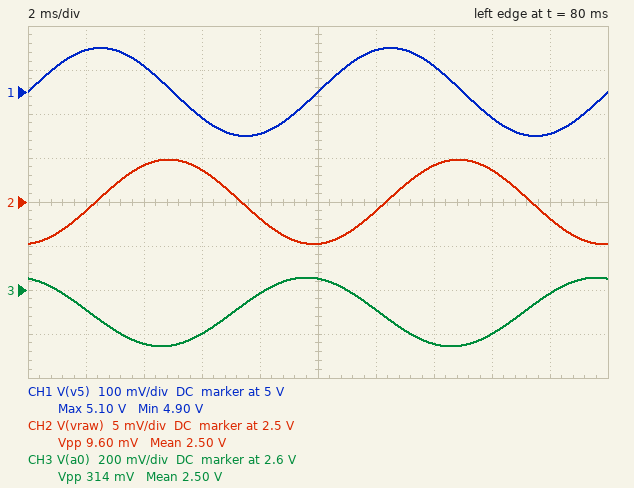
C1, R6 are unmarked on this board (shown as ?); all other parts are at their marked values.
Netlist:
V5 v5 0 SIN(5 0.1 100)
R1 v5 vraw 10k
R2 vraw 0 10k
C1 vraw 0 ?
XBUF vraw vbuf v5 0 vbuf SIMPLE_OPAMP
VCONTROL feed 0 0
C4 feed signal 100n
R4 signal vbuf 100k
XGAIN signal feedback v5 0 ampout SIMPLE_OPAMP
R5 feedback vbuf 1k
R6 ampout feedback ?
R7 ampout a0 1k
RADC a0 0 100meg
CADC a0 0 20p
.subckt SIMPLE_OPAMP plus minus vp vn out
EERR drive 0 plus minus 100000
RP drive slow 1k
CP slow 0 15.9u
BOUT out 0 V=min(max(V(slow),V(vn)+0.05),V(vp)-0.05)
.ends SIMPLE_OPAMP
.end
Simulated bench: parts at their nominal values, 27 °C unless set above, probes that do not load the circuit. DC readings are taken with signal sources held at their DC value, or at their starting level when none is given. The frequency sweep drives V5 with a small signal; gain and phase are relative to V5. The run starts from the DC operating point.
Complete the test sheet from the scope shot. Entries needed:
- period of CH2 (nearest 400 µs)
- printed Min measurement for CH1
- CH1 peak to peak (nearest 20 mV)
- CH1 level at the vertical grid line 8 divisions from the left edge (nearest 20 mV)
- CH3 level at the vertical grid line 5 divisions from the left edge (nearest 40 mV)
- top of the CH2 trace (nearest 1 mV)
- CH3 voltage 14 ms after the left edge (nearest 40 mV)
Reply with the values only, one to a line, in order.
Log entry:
10.0 ms
4.90 V
200 mV
4.94 V
2.64 V
2.505 V
2.36 V
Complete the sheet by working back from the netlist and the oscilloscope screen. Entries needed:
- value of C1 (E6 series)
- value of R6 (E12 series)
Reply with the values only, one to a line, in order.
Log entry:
3.3 µF
33 kΩ
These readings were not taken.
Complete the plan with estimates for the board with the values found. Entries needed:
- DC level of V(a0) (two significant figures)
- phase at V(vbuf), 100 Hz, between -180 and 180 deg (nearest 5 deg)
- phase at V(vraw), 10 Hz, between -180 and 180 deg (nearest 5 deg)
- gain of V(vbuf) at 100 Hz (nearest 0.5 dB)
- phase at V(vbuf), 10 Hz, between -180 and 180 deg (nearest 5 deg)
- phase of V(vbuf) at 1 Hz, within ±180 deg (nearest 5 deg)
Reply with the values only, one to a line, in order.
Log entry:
2.5 V
-85 deg
-45 deg
-26.5 dB
-45 deg
-5 deg
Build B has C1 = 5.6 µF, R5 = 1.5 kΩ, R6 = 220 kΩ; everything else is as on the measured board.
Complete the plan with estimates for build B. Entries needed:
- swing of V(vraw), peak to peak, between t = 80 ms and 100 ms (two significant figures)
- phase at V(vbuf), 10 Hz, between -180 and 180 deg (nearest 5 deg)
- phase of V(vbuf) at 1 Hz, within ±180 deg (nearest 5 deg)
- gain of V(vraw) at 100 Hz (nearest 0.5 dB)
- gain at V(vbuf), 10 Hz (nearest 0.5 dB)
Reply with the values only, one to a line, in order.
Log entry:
5.7 mV
-60 deg
-10 deg
-31.0 dB
-12.0 dB
